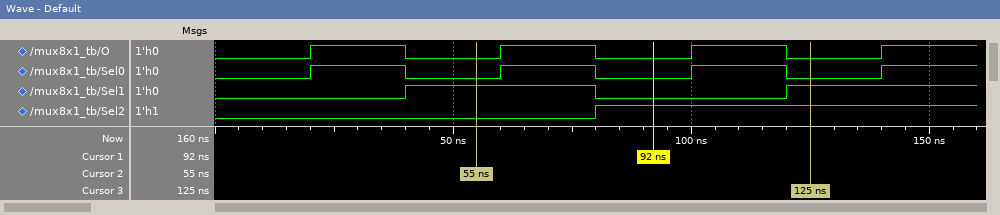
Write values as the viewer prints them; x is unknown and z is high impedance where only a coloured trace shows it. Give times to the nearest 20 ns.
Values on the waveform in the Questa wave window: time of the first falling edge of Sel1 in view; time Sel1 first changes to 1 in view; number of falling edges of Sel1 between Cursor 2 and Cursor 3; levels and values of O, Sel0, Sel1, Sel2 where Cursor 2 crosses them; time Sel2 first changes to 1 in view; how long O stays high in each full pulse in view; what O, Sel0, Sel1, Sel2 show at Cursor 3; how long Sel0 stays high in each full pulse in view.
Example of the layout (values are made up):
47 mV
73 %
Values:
80 ns
40 ns
1
O=0, Sel0=0, Sel1=1, Sel2=0
80 ns
20 ns, 20 ns, 20 ns
O=0, Sel0=0, Sel1=1, Sel2=1
20 ns, 20 ns, 20 ns
